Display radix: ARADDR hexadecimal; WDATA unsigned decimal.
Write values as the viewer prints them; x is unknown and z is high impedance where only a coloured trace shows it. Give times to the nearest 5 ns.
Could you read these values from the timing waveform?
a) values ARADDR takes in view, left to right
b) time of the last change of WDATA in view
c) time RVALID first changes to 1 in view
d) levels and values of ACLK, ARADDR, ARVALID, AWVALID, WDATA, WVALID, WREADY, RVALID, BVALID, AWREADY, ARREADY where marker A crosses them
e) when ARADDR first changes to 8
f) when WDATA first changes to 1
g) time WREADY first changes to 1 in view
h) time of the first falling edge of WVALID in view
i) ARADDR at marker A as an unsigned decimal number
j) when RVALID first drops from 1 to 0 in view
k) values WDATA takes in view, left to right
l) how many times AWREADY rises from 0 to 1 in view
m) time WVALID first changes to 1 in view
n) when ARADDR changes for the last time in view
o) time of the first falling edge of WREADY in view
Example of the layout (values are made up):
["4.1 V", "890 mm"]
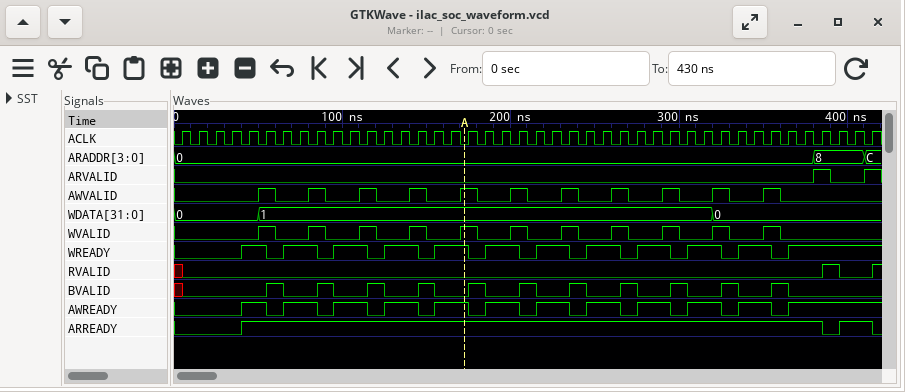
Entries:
["0, 8, C", "320 ns", "385 ns", "ACLK=0, ARADDR=0, ARVALID=0, AWVALID=1, WDATA=1, WVALID=1, WREADY=1, RVALID=0, BVALID=0, AWREADY=1, ARREADY=1", "380 ns", "50 ns", "40 ns", "60 ns", "0", "395 ns", "0, 1, 0", "12", "50 ns", "410 ns", "55 ns"]
